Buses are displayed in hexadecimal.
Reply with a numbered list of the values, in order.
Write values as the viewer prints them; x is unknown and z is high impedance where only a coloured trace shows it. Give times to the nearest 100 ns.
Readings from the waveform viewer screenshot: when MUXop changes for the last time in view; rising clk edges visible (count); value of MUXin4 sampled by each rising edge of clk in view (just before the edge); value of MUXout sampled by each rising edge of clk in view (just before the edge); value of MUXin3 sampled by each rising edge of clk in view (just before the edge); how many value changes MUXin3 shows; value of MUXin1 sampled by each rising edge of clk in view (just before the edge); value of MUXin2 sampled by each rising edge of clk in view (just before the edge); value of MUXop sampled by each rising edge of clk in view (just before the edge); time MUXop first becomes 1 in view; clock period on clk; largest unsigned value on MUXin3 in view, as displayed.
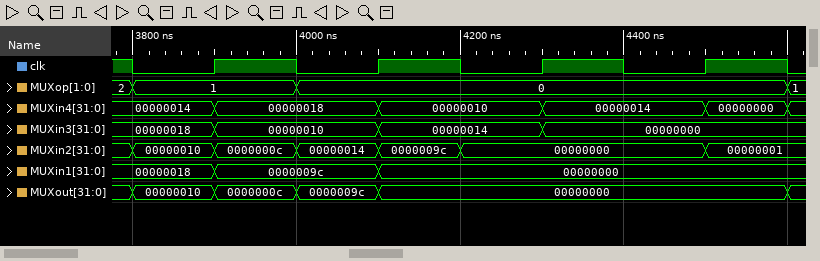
1. 4600 ns
2. 4
3. 00000014, 00000018, 00000010, 00000014
4. 00000010, 0000009c, 00000000, 00000000
5. 00000018, 00000010, 00000014, 00000000
6. 3
7. 00000018, 0000009c, 00000000, 00000000
8. 00000010, 00000014, 00000000, 00000000
9. 1, 0, 0, 0
10. 3800 ns
11. 200 ns
12. 00000018
